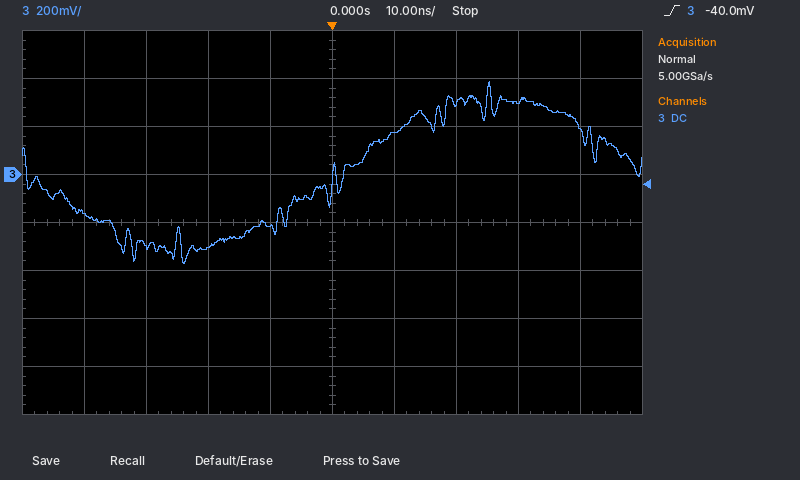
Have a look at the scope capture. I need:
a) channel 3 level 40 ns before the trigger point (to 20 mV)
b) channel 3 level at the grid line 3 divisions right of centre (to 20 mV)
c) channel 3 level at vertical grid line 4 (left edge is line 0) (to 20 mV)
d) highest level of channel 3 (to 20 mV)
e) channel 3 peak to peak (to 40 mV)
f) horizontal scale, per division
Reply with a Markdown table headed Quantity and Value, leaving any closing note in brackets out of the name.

| Quantity | Value |
|---|---|
| channel 3 level 40 ns before the trigger point | -160 mV |
| channel 3 level at the grid line 3 divisions right of centre | 300 mV |
| channel 3 level at vertical grid line 4 (left edge is line 0) | -220 mV |
| highest level of channel 3 | 380 mV |
| channel 3 peak to peak | 760 mV |
| horizontal scale, per division | 10 ns |
